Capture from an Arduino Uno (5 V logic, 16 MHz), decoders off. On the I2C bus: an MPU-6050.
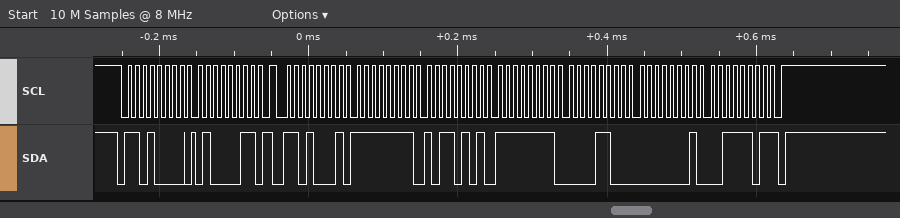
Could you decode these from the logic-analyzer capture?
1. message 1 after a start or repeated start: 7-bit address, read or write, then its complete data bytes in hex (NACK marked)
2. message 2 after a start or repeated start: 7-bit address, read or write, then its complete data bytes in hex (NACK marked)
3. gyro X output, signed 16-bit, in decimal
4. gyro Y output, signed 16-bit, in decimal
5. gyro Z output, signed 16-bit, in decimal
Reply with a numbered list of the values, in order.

1. 0x68 write: 43
2. 0x68 read: FF B5 FF 0C 01 3D NACK
3. -75
4. -244
5. 317
